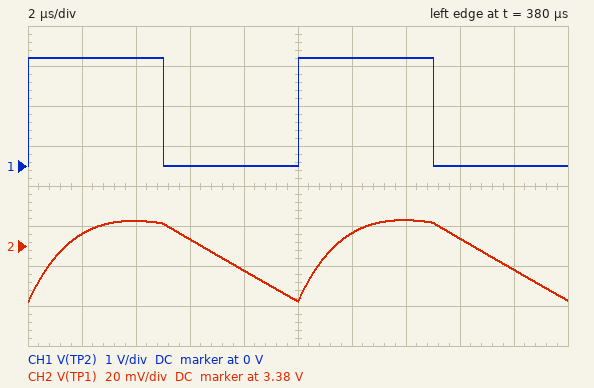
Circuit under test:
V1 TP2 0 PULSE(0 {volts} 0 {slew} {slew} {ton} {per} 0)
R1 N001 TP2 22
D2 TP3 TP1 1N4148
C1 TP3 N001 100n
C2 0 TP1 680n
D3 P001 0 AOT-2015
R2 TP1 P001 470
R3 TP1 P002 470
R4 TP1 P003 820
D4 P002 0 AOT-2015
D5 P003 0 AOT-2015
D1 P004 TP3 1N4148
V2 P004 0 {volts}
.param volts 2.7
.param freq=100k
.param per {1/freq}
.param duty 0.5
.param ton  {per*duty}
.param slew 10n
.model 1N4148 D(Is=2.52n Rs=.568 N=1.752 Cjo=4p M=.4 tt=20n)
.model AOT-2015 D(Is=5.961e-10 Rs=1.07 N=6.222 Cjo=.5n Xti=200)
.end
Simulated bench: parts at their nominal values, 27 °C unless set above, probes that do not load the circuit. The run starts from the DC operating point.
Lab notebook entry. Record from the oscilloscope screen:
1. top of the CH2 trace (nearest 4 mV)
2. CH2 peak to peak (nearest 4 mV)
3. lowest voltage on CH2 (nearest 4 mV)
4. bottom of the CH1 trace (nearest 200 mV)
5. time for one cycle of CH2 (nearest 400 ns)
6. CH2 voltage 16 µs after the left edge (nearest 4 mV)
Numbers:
3.392 V
40 mV
3.352 V
0 V
10.0 µs
3.384 V
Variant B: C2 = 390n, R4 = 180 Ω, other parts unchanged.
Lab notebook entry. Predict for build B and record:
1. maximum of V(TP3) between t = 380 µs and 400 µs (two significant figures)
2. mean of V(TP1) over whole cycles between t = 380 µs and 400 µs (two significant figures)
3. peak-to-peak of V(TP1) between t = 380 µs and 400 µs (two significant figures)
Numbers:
3.9 V
3.2 V
91 mV
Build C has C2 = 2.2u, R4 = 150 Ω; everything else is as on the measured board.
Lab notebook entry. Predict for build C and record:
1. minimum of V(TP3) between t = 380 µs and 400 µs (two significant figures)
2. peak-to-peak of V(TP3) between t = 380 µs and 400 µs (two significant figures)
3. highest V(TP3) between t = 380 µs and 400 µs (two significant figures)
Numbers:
1.9 V
1.9 V
3.8 V
